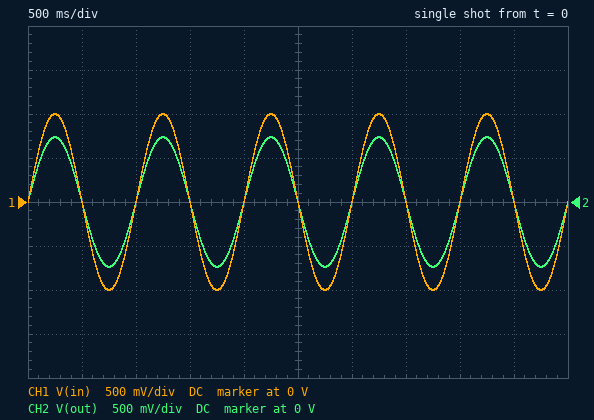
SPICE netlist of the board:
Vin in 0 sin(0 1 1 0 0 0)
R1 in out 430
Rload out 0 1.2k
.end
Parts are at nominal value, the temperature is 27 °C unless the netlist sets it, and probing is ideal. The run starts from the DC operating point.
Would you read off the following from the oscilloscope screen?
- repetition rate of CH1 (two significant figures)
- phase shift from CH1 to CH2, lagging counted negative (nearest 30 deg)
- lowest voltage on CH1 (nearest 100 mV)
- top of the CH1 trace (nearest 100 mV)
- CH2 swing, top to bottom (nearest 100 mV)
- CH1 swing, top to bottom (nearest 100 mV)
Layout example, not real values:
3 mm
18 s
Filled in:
1.0 Hz
0 deg
-1.0 V
1.0 V
1.5 V
2.0 V
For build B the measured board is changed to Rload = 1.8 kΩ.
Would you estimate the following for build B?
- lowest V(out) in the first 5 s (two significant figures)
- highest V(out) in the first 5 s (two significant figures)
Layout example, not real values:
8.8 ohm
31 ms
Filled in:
-810 mV
810 mV
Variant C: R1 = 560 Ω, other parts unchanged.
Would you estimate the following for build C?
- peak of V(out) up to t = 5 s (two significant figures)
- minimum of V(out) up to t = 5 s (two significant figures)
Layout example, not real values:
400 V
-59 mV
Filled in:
680 mV
-680 mV
